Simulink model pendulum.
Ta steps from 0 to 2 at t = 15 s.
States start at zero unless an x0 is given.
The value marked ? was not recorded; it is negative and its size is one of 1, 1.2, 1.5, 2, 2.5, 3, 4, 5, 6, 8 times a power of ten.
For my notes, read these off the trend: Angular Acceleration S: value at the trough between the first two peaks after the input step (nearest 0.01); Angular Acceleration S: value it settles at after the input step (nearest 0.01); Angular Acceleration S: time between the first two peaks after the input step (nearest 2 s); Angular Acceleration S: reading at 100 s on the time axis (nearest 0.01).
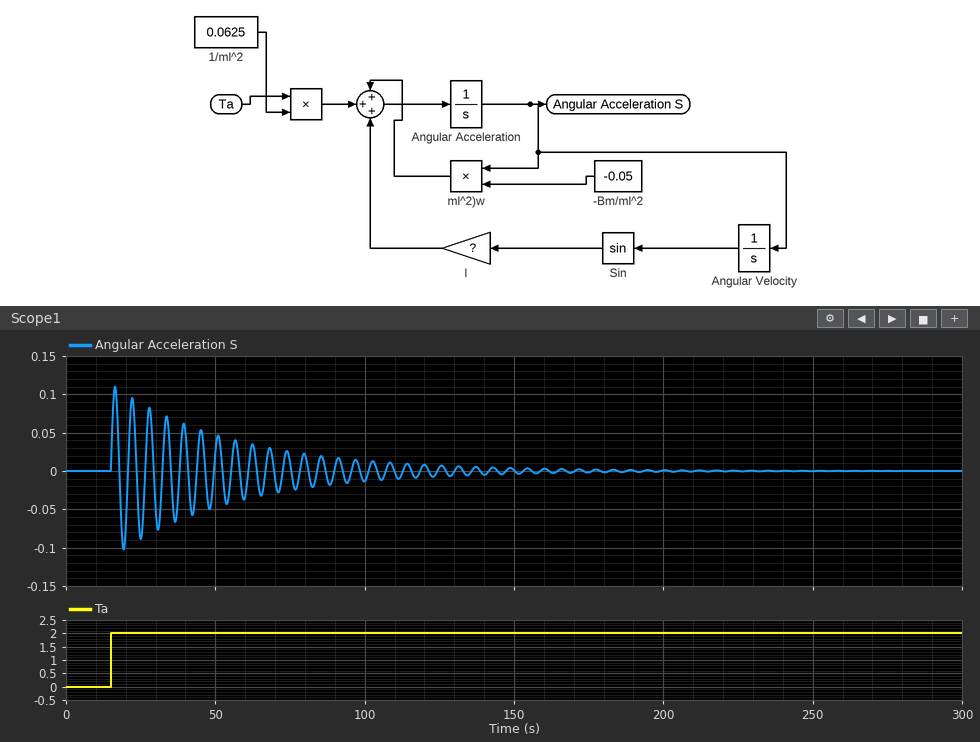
-0.10
0.00
6 s
-0.01
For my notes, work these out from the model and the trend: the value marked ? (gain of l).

-1.2
